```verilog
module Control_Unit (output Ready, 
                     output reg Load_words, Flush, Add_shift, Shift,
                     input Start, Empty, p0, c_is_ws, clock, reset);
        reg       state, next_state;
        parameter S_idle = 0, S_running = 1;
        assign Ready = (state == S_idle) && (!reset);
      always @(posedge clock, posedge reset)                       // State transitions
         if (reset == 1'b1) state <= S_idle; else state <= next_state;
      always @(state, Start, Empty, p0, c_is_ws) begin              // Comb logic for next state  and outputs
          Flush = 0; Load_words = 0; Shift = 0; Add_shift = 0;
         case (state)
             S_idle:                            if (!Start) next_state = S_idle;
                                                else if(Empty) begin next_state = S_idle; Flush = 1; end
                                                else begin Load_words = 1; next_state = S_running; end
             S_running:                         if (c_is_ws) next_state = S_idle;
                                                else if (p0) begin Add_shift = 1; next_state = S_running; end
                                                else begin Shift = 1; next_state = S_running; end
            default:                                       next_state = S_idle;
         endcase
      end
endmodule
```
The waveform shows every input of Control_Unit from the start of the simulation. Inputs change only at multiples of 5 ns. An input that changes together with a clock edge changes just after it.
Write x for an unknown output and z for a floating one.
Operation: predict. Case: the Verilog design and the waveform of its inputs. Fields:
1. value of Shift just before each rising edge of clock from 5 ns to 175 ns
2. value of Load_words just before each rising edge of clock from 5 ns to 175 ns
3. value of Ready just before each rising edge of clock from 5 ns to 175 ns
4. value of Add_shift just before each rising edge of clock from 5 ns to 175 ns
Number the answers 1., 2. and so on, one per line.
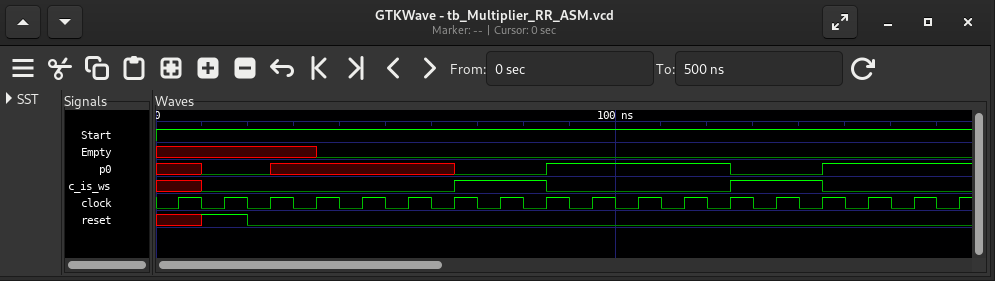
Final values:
1. 0 0 0 1 1 1 1 0 0 0 0 0 0 0 0 0 0 0
2. 0 1 1 0 0 0 0 0 1 0 0 0 0 0 1 0 0 0
3. x 0 1 0 0 0 0 0 1 0 0 0 0 0 1 0 0 0
4. 0 0 0 0 0 0 0 0 0 1 1 1 1 0 0 1 1 1
